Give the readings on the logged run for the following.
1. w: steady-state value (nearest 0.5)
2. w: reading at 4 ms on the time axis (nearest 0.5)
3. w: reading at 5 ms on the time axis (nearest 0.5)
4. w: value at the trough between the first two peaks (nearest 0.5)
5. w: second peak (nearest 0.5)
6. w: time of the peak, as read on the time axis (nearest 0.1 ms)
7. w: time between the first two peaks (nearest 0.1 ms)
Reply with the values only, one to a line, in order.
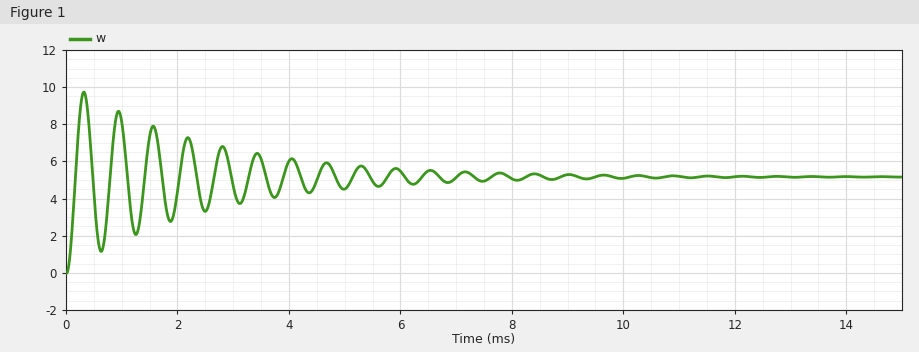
5.0
6.0
4.5
1.0
8.5
0.3 ms
0.6 ms
